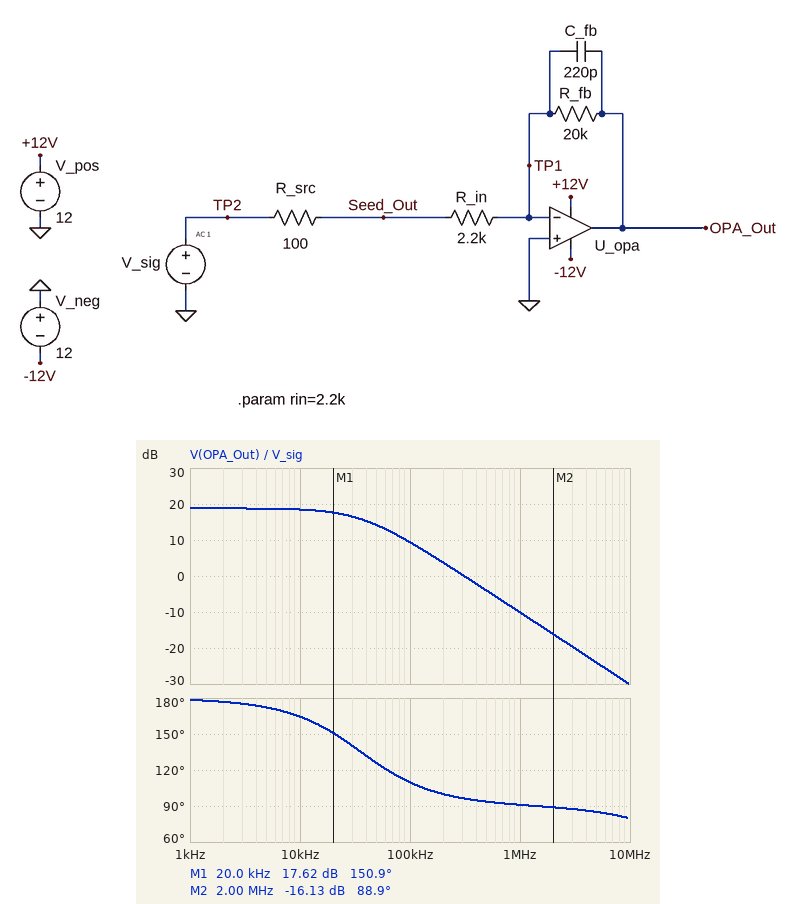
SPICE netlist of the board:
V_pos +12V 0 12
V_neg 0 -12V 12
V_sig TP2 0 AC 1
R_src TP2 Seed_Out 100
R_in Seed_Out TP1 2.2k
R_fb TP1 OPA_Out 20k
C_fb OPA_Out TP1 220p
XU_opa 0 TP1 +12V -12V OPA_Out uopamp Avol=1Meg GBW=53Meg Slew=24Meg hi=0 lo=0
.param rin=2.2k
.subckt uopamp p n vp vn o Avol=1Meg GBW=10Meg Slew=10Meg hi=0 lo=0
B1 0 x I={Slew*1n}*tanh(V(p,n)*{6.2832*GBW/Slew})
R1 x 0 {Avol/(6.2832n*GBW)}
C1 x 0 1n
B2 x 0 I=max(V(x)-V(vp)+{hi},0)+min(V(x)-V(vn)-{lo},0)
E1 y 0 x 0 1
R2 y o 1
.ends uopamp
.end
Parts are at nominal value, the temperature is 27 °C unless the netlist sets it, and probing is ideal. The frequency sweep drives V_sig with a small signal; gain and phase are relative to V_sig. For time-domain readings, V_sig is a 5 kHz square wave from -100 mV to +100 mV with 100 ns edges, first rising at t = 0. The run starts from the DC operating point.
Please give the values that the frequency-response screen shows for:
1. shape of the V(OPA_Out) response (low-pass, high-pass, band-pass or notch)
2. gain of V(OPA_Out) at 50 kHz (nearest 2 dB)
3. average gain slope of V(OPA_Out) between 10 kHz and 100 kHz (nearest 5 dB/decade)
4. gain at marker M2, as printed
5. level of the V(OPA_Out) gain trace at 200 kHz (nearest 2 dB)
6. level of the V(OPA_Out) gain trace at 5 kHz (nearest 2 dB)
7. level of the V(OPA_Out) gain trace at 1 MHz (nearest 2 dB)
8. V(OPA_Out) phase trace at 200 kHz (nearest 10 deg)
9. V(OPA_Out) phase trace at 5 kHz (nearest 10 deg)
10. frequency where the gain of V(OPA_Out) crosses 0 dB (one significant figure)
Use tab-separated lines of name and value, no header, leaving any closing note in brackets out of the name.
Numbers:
shape of the V(OPA_Out) response	low-pass
gain of V(OPA_Out) at 50 kHz	14 dB
average gain slope of V(OPA_Out) between 10 kHz and 100 kHz	-10 dB/decade
gain at marker M2, as printed	-16.13 dB
level of the V(OPA_Out) gain trace at 200 kHz	4 dB
level of the V(OPA_Out) gain trace at 5 kHz	18 dB
level of the V(OPA_Out) gain trace at 1 MHz	-10 dB
V(OPA_Out) phase trace at 200 kHz	100 deg
V(OPA_Out) phase trace at 5 kHz	170 deg
frequency where the gain of V(OPA_Out) crosses 0 dB	300 kHz
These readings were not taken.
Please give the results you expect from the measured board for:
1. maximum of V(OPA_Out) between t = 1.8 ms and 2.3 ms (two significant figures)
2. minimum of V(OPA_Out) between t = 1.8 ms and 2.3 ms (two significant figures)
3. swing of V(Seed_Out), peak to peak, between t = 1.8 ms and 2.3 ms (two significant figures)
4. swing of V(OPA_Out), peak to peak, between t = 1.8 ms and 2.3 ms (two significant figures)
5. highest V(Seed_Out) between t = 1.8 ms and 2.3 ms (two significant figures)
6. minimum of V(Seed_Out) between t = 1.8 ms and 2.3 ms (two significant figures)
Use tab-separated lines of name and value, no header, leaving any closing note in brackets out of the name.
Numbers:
maximum of V(OPA_Out) between t = 1.8 ms and 2.3 ms	870 mV
minimum of V(OPA_Out) between t = 1.8 ms and 2.3 ms	-870 mV
swing of V(Seed_Out), peak to peak, between t = 1.8 ms and 2.3 ms	190 mV
swing of V(OPA_Out), peak to peak, between t = 1.8 ms and 2.3 ms	1.7 V
highest V(Seed_Out) between t = 1.8 ms and 2.3 ms	96 mV
minimum of V(Seed_Out) between t = 1.8 ms and 2.3 ms	-96 mV
